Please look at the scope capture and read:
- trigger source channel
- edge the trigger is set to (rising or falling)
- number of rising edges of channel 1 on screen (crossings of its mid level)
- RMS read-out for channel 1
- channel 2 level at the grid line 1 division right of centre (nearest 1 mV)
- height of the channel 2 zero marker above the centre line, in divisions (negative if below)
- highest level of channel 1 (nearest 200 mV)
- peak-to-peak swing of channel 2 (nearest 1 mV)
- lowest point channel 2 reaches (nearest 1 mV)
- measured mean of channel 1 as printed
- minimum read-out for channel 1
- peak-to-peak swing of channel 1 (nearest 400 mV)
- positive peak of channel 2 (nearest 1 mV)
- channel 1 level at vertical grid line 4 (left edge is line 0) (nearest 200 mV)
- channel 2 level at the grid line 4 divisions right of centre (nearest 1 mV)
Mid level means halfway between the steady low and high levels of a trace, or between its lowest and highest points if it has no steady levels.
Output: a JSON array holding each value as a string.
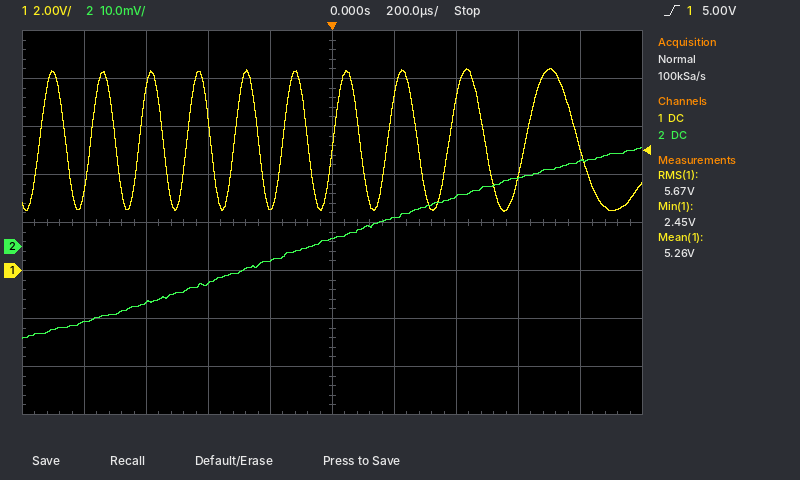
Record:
["channel 1", "rising", "10", "5.67 V", "6 mV", "-0.5 div", "8.4 V", "40 mV", "-19 mV", "5.26 V", "2.45 V", "6.0 V", "21 mV", "2.6 V", "18 mV"]
